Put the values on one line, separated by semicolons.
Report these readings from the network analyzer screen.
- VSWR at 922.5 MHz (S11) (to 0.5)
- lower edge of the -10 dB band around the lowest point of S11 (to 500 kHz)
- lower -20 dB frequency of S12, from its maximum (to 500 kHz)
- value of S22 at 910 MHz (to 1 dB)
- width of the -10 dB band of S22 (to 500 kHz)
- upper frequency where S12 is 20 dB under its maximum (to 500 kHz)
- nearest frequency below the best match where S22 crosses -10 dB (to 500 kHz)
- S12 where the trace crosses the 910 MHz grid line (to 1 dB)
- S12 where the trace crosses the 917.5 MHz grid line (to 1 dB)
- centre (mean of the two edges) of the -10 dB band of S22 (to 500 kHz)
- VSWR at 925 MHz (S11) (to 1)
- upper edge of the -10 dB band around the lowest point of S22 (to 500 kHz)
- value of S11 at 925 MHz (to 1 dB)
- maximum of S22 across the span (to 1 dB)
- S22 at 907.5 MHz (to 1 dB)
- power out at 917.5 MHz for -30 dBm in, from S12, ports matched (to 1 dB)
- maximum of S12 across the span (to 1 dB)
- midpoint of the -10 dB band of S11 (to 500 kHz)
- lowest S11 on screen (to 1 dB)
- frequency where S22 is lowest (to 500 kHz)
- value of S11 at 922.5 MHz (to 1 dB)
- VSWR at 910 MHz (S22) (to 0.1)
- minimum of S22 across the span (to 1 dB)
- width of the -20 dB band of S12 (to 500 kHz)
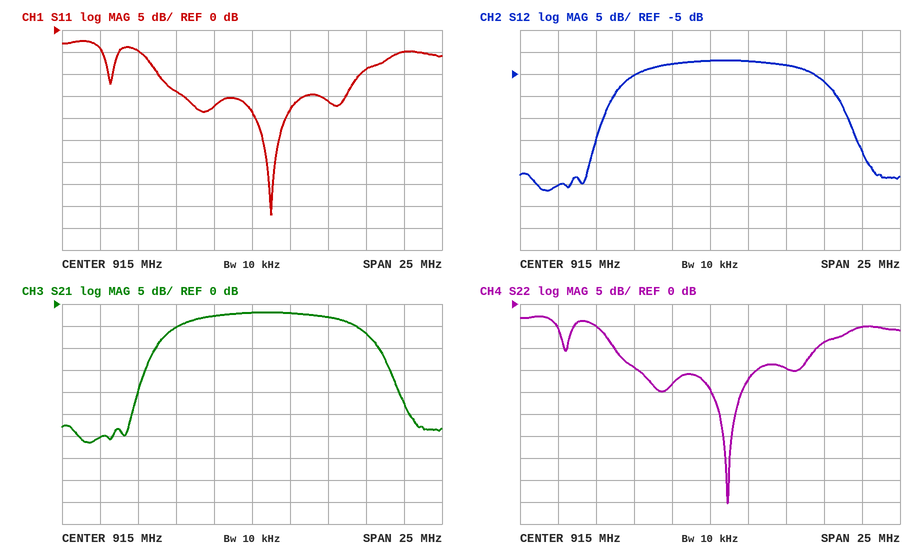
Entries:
2.0; 909.0 MHz; 907.5 MHz; -14 dB; 13.5 MHz; 925.0 MHz; 908.5 MHz; -5 dB; -2 dB; 915.5 MHz; 4; 922.0 MHz; -5 dB; -3 dB; -5 dB; -32 dBm; -2 dB; 915.5 MHz; -42 dB; 916.0 MHz; -9 dB; 1.5; -45 dB; 17.5 MHz
